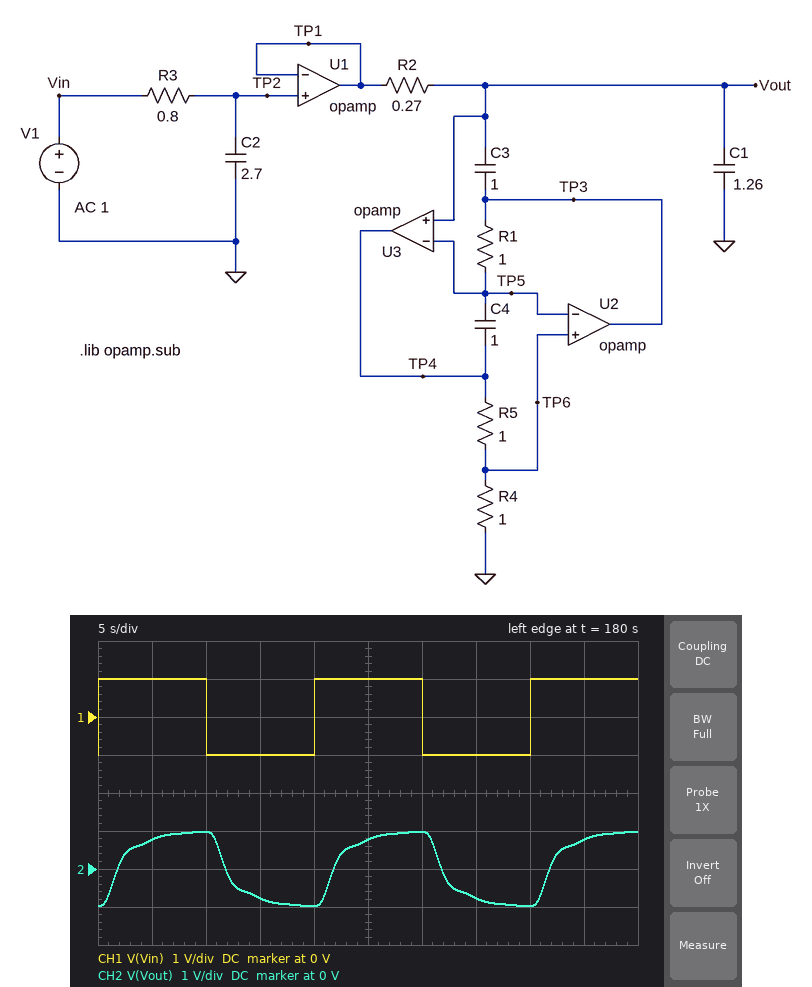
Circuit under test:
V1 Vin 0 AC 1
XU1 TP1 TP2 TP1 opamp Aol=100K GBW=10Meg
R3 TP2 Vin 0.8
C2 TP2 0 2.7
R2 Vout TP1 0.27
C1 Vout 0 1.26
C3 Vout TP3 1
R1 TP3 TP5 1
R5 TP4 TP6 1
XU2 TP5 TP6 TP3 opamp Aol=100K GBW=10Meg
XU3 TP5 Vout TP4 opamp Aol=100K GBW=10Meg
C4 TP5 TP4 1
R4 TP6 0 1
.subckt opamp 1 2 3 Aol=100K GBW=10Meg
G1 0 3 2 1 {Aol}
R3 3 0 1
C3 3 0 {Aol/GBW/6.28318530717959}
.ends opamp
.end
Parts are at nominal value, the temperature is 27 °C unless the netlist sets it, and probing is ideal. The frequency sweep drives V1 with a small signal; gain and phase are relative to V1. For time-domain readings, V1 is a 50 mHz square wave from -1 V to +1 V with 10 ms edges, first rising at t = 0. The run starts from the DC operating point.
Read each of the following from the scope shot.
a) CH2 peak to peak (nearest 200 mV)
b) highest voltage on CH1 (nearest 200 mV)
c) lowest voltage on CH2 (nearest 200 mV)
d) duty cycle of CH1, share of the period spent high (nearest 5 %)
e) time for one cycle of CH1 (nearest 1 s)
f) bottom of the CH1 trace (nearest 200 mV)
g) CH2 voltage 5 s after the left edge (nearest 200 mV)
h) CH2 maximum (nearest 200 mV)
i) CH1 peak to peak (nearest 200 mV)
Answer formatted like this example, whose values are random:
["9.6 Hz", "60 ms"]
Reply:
["2.0 V", "1.0 V", "-1.0 V", "50 %", "20 s", "-1.0 V", "800 mV", "1.0 V", "2.0 V"]
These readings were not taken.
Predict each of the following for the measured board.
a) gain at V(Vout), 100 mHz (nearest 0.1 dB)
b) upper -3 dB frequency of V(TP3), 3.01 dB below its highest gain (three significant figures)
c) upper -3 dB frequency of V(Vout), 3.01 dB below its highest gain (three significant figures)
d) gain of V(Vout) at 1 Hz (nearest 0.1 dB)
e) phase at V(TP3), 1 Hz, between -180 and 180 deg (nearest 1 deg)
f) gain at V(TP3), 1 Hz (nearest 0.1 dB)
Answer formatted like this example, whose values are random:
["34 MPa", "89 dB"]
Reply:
["-3.8 dB", "326 mHz", "82.1 mHz", "-42.6 dB", "26 deg", "-26.5 dB"]
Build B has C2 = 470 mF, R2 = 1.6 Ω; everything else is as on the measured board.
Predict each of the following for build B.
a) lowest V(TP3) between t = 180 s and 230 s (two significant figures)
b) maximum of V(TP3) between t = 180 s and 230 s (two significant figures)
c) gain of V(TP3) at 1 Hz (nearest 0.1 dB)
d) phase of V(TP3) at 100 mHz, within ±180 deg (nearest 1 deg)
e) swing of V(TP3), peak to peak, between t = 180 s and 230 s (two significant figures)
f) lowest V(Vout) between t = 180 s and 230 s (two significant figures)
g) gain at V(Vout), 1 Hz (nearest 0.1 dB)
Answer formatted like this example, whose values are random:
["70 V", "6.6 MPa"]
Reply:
["-1.3 V", "1.3 V", "-28.2 dB", "-119 deg", "2.5 V", "-1.0 V", "-44.2 dB"]
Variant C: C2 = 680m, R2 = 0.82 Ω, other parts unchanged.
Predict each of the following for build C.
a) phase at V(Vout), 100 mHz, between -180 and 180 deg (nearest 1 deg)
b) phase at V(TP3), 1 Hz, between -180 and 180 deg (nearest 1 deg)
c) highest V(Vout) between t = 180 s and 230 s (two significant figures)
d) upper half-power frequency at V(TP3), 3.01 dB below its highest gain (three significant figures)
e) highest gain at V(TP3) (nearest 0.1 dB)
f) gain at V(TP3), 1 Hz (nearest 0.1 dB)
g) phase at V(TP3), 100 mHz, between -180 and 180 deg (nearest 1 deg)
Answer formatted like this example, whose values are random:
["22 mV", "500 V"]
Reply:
["-63 deg", "37 deg", "1.2 V", "223 mHz", "1.8 dB", "-25.1 dB", "-95 deg"]
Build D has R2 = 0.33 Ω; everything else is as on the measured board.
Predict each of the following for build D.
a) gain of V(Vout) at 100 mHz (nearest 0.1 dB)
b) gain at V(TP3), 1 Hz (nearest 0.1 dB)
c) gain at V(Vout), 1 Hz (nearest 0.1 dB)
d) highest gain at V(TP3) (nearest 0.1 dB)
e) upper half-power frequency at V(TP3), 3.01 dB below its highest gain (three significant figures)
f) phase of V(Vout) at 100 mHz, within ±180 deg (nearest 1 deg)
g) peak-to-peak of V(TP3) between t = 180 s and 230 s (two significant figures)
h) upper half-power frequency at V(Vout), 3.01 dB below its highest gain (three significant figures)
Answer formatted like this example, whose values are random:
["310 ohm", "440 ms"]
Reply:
["-3.7 dB", "-28.4 dB", "-44.5 dB", "0 dB", "279 mHz", "-70 deg", "2.7 V", "83.7 mHz"]
